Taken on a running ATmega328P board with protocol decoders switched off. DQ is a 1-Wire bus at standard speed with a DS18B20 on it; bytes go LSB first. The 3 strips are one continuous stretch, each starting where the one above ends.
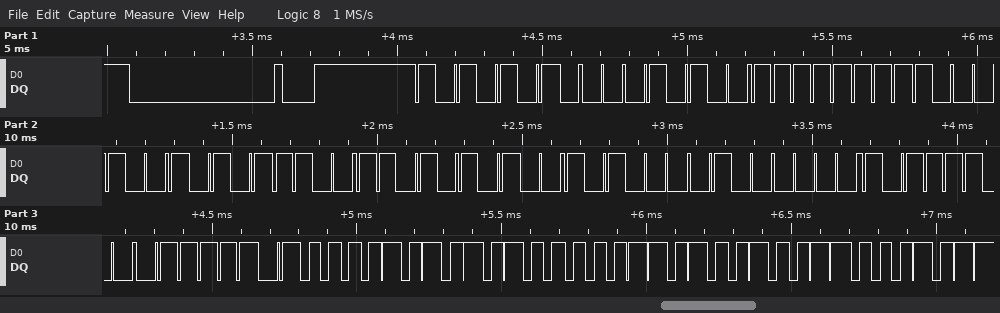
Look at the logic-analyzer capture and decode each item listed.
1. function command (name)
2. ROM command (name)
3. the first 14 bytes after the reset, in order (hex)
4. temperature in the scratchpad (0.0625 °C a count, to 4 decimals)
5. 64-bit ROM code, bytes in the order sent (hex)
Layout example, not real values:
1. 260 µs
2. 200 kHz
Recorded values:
1. Read Scratchpad
2. Match ROM
3. 55 28 FF 91 3A AB 14 02 3D BE 50 05 4B 46
4. 85.0000 °C
5. 28 FF 91 3A AB 14 02 3D
